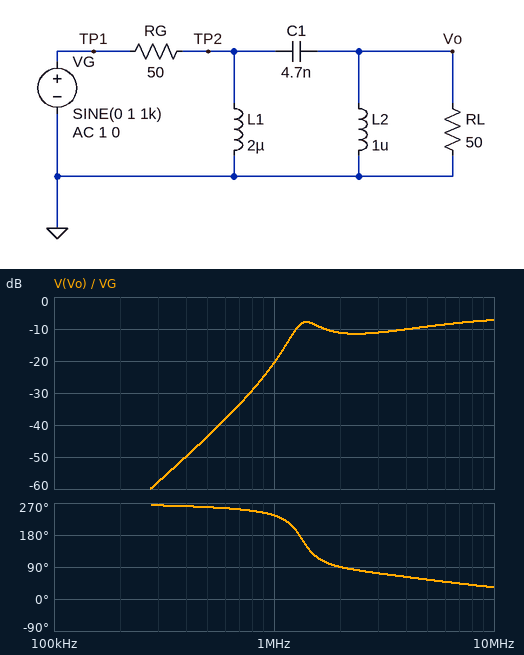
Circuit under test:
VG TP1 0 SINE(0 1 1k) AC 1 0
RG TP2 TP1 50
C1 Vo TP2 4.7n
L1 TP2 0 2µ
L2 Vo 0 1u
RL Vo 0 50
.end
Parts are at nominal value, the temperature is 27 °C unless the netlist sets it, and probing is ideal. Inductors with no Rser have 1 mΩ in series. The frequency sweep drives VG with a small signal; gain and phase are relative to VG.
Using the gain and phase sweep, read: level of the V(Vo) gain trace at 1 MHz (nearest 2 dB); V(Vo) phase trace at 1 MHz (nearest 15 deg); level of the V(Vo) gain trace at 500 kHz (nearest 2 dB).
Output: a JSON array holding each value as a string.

["-20 dB", "240 deg", "-44 dB"]
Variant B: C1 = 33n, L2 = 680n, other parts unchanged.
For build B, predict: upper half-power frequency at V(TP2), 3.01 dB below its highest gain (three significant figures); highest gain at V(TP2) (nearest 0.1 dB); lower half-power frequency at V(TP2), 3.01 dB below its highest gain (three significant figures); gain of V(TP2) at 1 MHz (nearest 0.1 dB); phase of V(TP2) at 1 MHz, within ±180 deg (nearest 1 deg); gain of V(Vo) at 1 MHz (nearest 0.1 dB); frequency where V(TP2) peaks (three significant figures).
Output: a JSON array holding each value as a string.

["564 kHz", "-1.0 dB", "504 kHz", "-36.9 dB", "-56 deg", "-21.1 dB", "534 kHz"]
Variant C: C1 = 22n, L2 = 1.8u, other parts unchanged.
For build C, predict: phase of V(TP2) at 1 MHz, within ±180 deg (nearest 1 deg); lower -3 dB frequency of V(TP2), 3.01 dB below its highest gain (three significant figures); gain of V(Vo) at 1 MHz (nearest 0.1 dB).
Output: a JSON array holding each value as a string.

["61 deg", "508 kHz", "-15.6 dB"]
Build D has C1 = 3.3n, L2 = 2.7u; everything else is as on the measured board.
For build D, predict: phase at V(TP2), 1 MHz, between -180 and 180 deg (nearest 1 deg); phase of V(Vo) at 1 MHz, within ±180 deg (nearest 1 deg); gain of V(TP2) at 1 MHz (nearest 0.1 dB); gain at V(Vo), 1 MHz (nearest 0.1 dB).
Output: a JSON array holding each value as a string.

["64 deg", "-144 deg", "-8.9 dB", "-15.3 dB"]
